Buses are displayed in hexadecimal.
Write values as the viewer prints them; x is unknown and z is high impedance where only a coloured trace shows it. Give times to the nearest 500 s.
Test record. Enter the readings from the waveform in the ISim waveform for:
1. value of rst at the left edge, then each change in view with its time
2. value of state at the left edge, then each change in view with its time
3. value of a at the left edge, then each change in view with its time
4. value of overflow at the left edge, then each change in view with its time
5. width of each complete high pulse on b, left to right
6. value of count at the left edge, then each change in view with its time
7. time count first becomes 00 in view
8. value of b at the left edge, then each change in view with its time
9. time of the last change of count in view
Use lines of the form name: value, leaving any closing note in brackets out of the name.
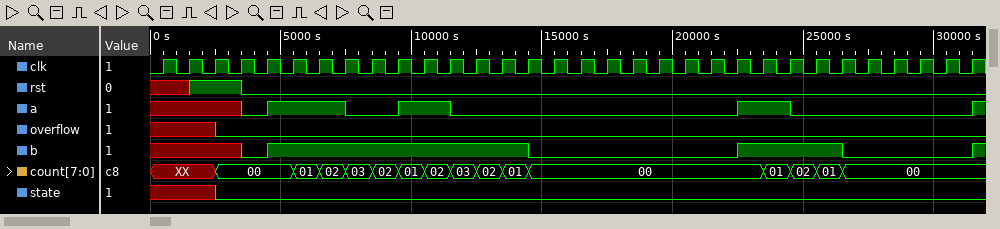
value of rst at the left edge, then each change in view with its time: x, 1 at 1500 s, 0 at 3500 s
value of state at the left edge, then each change in view with its time: x, 0 at 2500 s
value of a at the left edge, then each change in view with its time: x, 0 at 3500 s, 1 at 4500 s, 0 at 7500 s, 1 at 9500 s, 0 at 11500 s, 1 at 22500 s, 0 at 24500 s, 1 at 31500 s
value of overflow at the left edge, then each change in view with its time: x, 0 at 2500 s
width of each complete high pulse on b, left to right: 10000 s, 4000 s
value of count at the left edge, then each change in view with its time: XX, 00 at 2500 s, 01 at 5500 s, 02 at 6500 s, 03 at 7500 s, 02 at 8500 s, 01 at 9500 s, 02 at 10500 s, 03 at 11500 s, 02 at 12500 s, 01 at 13500 s, 00 at 14500 s, 01 at 23500 s, 02 at 24500 s, 01 at 25500 s, 00 at 26500 s
time count first becomes 00 in view: 2500 s
value of b at the left edge, then each change in view with its time: x, 0 at 3500 s, 1 at 4500 s, 0 at 14500 s, 1 at 22500 s, 0 at 26500 s, 1 at 31500 s
time of the last change of count in view: 26500 s
